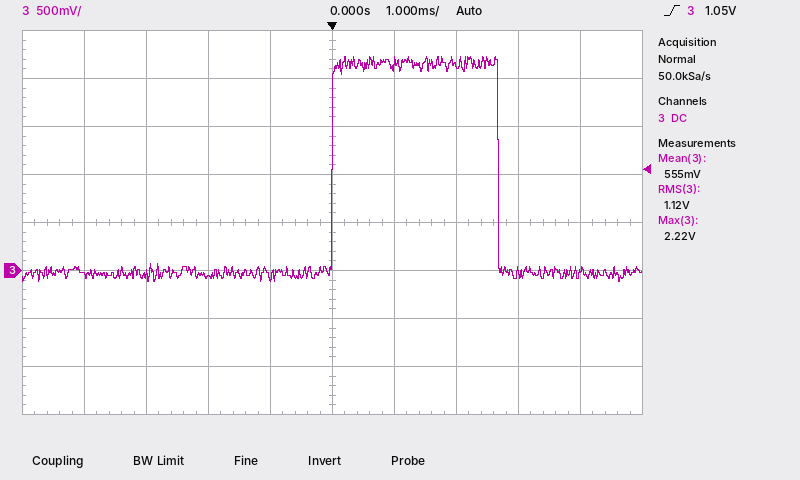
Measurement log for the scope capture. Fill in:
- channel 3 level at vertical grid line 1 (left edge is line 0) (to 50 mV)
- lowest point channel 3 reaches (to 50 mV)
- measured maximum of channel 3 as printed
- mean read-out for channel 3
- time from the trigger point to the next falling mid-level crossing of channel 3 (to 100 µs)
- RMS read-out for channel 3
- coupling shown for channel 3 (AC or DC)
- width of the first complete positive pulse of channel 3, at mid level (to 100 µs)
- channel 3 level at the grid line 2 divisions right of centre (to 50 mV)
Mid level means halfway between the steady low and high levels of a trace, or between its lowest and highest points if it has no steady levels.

-50 mV
-100 mV
2.22 V
555 mV
2.7 ms
1.12 V
DC
2.7 ms
2.15 V
